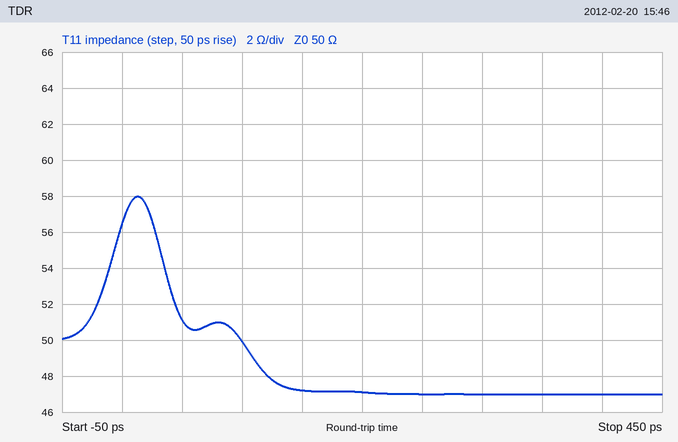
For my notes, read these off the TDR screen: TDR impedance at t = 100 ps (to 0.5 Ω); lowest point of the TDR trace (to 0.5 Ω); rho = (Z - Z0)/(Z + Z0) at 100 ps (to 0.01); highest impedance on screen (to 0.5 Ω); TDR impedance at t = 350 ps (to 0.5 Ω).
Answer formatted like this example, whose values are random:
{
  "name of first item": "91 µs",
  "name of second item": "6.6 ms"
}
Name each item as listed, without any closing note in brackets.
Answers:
{
  "TDR impedance at t = 100 ps": "50.0 Ω",
  "lowest point of the TDR trace": "47.0 Ω",
  "rho = (Z - Z0)/(Z + Z0) at 100 ps": "0.00",
  "highest impedance on screen": "58.0 Ω",
  "TDR impedance at t = 350 ps": "47.0 Ω"
}
